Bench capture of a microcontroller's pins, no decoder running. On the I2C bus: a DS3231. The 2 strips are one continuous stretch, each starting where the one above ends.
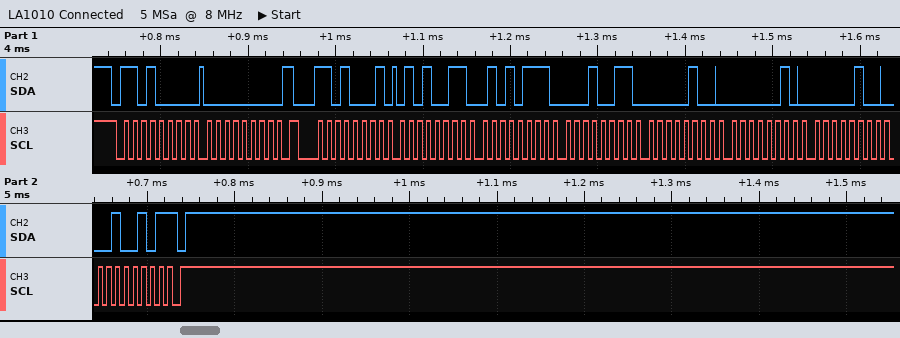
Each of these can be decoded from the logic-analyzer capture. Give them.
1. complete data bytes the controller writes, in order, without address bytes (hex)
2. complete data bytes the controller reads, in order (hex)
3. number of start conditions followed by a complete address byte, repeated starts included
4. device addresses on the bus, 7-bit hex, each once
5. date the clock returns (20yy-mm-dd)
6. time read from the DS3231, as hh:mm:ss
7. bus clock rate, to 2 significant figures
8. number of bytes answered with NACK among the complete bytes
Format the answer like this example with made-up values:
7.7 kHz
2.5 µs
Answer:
00
53 57 13 04 02 04 25
2
0x68
2025-04-02
13:57:53
100 kHz
1
